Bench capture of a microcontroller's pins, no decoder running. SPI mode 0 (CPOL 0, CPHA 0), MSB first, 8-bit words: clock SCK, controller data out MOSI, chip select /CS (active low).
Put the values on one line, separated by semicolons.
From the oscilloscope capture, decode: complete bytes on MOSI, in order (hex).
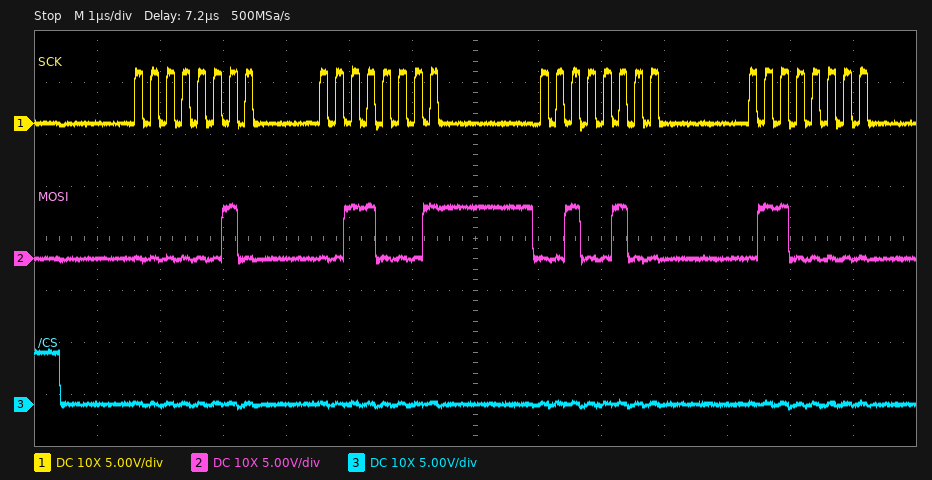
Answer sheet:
02 31 24 60
